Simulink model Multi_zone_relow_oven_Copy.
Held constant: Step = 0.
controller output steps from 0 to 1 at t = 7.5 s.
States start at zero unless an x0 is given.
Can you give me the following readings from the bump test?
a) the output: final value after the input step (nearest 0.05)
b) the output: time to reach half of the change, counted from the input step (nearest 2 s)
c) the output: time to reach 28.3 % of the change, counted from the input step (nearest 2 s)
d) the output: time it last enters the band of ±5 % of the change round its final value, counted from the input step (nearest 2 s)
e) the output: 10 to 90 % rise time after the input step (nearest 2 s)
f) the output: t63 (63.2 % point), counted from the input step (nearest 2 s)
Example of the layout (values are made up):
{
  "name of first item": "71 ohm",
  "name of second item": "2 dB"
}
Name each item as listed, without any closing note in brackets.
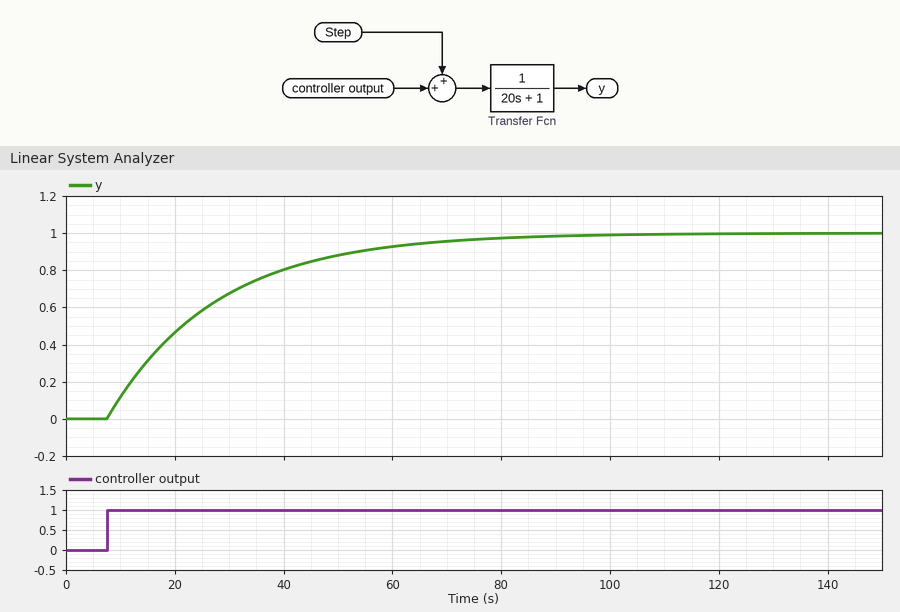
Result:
{
  "the output: final value after the input step": "1.00",
  "the output: time to reach half of the change, counted from the input step": "14 s",
  "the output: time to reach 28.3 % of the change, counted from the input step": "6 s",
  "the output: time it last enters the band of ±5 % of the change round its final value, counted from the input step": "60 s",
  "the output: 10 to 90 % rise time after the input step": "44 s",
  "the output: t63 (63.2 % point), counted from the input step": "20 s"
}
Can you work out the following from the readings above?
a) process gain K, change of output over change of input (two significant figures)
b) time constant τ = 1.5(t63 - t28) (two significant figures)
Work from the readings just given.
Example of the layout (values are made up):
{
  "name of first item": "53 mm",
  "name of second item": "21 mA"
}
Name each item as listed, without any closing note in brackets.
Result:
{
  "process gain K, change of output over change of input": "1.0",
  "time constant τ = 1.5(t63 - t28)": "21 s"
}
